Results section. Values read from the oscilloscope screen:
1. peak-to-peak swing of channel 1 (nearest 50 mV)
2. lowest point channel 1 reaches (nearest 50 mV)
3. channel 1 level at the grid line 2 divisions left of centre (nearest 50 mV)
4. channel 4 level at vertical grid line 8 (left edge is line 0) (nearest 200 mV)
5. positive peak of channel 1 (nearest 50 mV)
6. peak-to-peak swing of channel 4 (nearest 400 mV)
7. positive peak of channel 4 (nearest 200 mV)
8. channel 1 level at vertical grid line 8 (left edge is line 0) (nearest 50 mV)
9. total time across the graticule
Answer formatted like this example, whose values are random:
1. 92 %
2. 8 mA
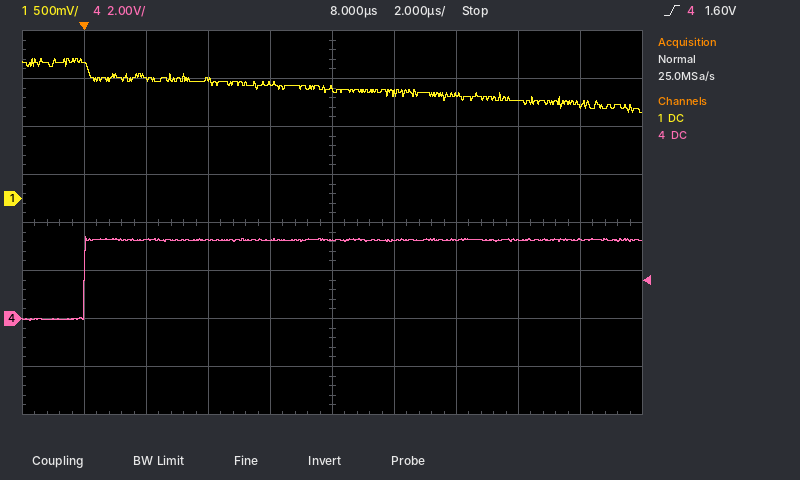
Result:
1. 550 mV
2. 900 mV
3. 1.25 V
4. 3.2 V
5. 1.45 V
6. 3.6 V
7. 3.4 V
8. 1.00 V
9. 20 µs
